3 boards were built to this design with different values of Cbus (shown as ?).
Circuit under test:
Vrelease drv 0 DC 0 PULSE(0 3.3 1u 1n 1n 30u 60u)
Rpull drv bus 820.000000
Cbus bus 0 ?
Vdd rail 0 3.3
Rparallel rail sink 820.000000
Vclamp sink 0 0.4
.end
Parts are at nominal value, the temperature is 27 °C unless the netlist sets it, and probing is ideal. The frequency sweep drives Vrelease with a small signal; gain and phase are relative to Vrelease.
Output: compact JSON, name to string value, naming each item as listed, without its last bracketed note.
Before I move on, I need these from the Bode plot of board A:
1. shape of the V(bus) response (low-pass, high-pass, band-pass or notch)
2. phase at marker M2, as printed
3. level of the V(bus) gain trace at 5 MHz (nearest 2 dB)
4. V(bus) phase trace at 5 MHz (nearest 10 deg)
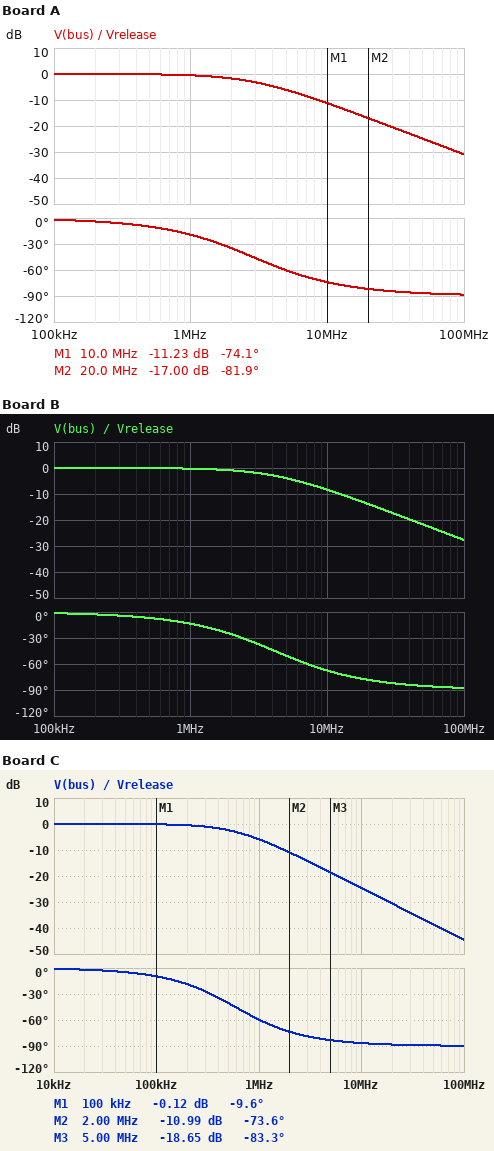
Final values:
{"shape of the V(bus) response": "low-pass", "phase at marker M2, as printed": "-81.9 deg", "level of the V(bus) gain trace at 5 MHz": "-6 dB", "V(bus) phase trace at 5 MHz": "-60 deg"}
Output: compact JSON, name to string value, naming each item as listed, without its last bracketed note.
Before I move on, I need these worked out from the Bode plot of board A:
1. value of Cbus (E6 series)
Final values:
{"value of Cbus": "68 pF"}
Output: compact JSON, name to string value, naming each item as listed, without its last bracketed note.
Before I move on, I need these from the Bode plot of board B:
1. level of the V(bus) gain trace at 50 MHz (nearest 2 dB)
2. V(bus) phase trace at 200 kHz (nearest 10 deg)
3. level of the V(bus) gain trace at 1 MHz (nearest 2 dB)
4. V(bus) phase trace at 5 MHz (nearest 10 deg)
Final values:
{"level of the V(bus) gain trace at 50 MHz": "-22 dB", "V(bus) phase trace at 200 kHz": "0 deg", "level of the V(bus) gain trace at 1 MHz": "0 dB", "V(bus) phase trace at 5 MHz": "-50 deg"}
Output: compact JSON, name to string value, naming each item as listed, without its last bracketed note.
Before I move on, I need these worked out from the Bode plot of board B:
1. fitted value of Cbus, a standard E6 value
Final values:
{"fitted value of Cbus, a standard E6 value": "47 pF"}
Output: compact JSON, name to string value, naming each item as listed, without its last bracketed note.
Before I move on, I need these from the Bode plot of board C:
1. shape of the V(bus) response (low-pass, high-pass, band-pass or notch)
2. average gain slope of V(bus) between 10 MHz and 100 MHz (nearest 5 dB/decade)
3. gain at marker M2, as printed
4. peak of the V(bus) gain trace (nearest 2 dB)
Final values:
{"shape of the V(bus) response": "low-pass", "average gain slope of V(bus) between 10 MHz and 100 MHz": "-20 dB/decade", "gain at marker M2, as printed": "-10.99 dB", "peak of the V(bus) gain trace": "0 dB"}
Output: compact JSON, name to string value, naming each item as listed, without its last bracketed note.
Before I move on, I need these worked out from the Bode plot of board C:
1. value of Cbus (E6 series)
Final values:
{"value of Cbus": "330 pF"}
